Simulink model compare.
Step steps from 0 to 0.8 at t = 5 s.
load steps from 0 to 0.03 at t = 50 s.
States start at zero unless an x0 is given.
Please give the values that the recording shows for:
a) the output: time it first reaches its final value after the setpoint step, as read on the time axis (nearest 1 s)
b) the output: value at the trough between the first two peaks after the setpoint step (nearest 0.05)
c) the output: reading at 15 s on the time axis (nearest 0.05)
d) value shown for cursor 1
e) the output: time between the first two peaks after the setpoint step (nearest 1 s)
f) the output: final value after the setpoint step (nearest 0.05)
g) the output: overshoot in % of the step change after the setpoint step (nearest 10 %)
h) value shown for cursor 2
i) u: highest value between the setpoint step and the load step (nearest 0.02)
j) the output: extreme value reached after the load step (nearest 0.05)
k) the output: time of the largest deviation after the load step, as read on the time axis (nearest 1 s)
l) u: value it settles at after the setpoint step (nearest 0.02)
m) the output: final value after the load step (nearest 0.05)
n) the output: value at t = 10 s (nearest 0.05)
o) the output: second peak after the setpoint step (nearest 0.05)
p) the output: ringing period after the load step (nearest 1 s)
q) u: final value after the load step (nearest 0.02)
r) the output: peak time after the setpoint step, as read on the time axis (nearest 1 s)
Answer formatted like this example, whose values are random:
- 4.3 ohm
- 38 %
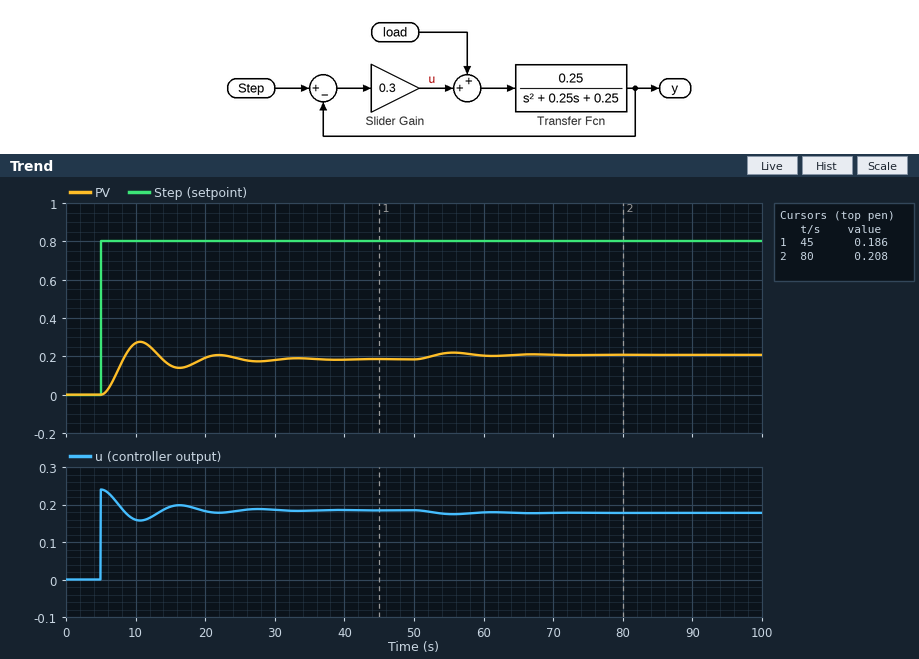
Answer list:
- 8 s
- 0.15
- 0.15
- 0.186
- 11 s
- 0.20
- 50 %
- 0.208
- 0.24
- 0.20
- 56 s
- 0.18
- 0.20
- 0.25
- 0.20
- 11 s
- 0.18
- 11 s
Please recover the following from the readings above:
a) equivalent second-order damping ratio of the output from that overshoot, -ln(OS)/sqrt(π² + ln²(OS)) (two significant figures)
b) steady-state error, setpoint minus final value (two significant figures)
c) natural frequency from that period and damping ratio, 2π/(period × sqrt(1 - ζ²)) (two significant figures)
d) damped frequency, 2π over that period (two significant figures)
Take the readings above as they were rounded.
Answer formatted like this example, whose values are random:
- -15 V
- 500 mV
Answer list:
- 0.22
- 0.60
- 0.59 rad/s
- 0.57 rad/s
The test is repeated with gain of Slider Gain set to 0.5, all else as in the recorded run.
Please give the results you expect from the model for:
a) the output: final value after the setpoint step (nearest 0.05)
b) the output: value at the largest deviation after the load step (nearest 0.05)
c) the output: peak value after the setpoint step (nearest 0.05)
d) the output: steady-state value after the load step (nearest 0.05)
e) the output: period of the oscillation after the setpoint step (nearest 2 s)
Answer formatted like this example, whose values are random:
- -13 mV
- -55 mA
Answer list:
- 0.25
- 0.30
- 0.40
- 0.30
- 10 s
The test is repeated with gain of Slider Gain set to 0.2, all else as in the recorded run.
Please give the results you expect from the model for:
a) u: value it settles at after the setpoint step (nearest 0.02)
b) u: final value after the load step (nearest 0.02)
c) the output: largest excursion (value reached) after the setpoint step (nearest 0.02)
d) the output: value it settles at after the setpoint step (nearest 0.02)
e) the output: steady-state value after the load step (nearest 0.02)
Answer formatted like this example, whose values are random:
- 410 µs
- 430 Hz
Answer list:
- 0.14
- 0.12
- 0.20
- 0.14
- 0.16
